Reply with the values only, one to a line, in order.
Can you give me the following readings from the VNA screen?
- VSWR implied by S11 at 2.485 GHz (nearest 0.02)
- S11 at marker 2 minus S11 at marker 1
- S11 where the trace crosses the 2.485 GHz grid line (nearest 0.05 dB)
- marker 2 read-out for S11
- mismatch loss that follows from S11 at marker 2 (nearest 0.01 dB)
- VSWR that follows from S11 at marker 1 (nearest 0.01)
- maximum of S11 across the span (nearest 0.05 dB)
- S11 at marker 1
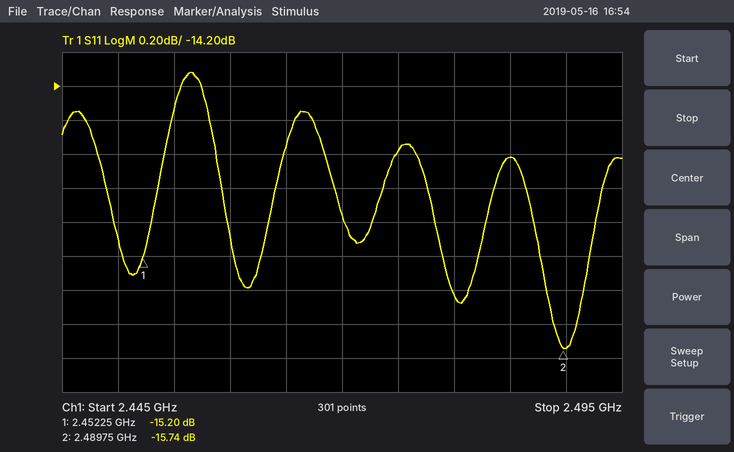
1.46
-0.54 dB
-14.60 dB
-15.74 dB
0.12 dB
1.42
-14.10 dB
-15.20 dB
